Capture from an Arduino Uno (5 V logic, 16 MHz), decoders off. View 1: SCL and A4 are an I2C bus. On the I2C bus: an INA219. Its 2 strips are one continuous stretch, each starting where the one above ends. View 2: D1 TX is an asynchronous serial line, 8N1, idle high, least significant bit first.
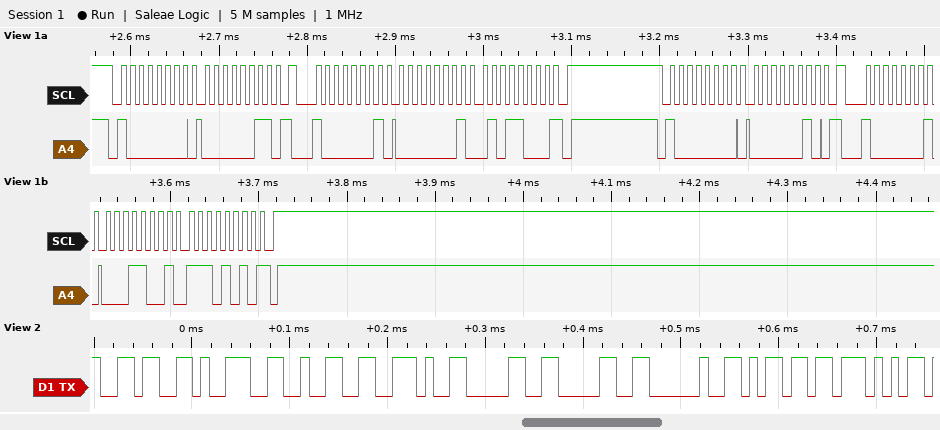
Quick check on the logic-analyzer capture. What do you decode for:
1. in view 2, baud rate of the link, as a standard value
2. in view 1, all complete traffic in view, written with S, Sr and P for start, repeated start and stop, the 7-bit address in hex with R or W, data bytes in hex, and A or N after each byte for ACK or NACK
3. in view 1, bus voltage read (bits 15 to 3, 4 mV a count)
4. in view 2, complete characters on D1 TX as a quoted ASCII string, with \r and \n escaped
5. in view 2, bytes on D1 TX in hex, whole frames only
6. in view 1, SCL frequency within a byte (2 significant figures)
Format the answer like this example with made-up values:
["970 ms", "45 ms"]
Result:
["115200 baud", "S 40W A 03 A Sr 40R A 01 A 58 N P S 40W A 02 A Sr 40R A 19 A EA N P", "3.316 V", "\"692.00 mW\"", "36 39 32 2E 30 30 20 6D 57", "100 kHz"]
